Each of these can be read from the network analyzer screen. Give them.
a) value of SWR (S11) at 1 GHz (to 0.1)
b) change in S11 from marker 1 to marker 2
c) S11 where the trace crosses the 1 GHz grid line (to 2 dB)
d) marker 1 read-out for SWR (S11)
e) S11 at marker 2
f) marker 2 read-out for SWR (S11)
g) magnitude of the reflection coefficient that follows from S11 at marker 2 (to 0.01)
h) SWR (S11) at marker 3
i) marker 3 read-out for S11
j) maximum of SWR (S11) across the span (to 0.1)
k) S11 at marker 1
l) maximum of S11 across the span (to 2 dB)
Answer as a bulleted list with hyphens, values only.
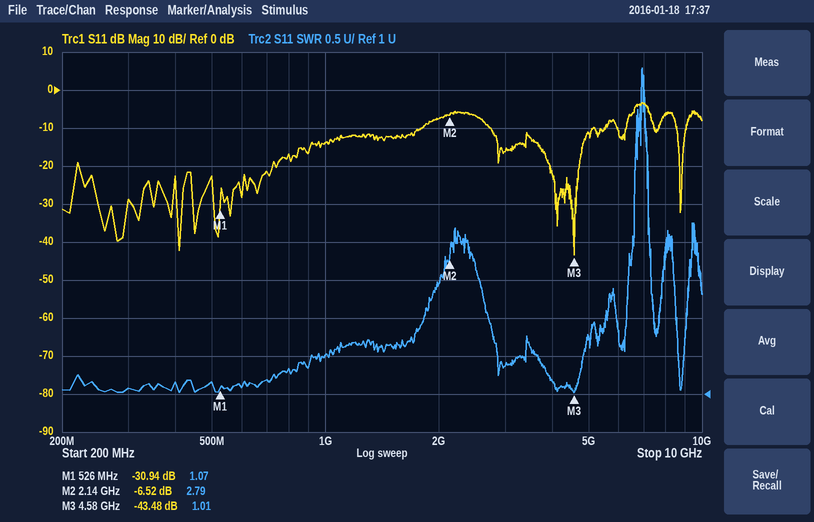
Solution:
- 1.5
- 24.42 dB
- -14 dB
- 1.07
- -6.52 dB
- 2.79
- 0.47
- 1.01
- -43.48 dB
- 5.3
- -30.94 dB
- -4 dB
